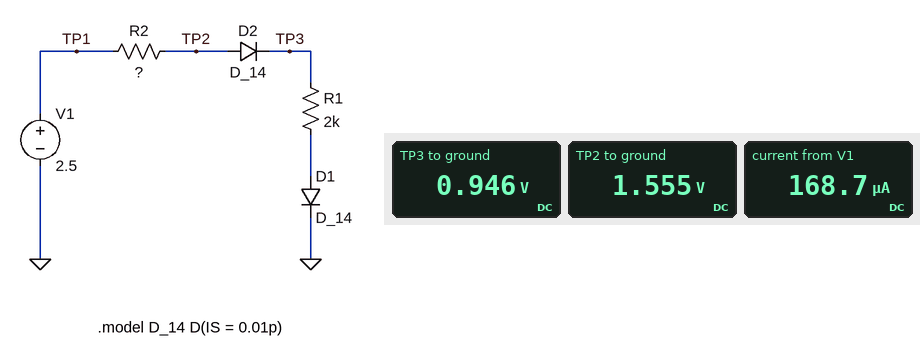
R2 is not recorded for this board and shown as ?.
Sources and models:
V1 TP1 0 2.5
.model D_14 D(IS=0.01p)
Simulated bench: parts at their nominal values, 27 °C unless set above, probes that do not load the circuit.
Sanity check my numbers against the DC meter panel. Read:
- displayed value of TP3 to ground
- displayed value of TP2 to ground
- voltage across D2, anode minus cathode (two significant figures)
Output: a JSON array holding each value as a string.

["0.946 V", "1.555 V", "610 mV"]
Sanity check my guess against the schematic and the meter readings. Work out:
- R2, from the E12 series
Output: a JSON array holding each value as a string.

["5.6 kΩ"]
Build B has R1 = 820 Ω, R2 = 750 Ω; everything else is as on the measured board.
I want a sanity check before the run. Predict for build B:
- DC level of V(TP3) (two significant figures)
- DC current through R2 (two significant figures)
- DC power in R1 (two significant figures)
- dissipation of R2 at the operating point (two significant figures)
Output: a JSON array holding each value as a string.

["1.3 V", "770 µA", "480 µW", "440 µW"]
